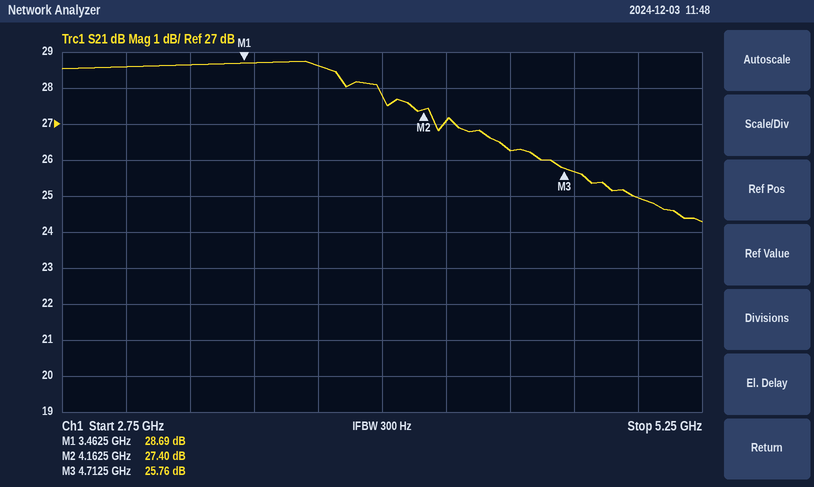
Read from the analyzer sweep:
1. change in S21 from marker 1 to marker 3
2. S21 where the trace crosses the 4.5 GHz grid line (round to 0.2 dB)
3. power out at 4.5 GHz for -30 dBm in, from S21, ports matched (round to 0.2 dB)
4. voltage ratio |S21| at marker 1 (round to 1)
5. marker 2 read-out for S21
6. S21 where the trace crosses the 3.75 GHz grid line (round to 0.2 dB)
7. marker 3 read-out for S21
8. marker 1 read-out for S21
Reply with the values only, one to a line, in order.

-2.93 dB
26.2 dB
-3.8 dBm
27
27.40 dB
28.6 dB
25.76 dB
28.69 dB
